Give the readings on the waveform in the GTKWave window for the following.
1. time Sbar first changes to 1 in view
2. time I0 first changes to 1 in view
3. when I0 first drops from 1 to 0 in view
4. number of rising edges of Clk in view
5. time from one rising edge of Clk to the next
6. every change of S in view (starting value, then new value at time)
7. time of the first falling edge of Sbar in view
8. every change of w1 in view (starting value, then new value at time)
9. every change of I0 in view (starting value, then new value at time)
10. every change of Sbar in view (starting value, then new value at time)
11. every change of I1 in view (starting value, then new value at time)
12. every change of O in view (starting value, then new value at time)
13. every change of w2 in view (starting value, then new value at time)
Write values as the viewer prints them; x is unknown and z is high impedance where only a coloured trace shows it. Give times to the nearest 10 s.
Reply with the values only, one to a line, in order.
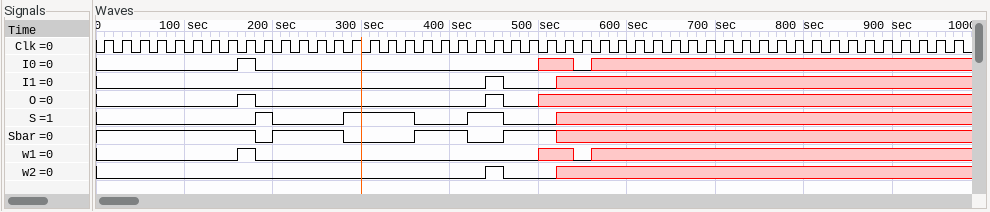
200 s
160 s
180 s
49
20 s
0, 1 at 180 s, 0 at 200 s, 1 at 280 s, 0 at 360 s, 1 at 420 s, 0 at 460 s, x at 520 s
180 s
0, 1 at 160 s, 0 at 180 s, x at 500 s, 0 at 540 s, x at 560 s
0, 1 at 160 s, 0 at 180 s, x at 500 s, 0 at 540 s, x at 560 s
1, 0 at 180 s, 1 at 200 s, 0 at 280 s, 1 at 360 s, 0 at 420 s, 1 at 460 s, x at 520 s
0, 1 at 440 s, 0 at 460 s, x at 520 s
0, 1 at 160 s, 0 at 180 s, 1 at 440 s, 0 at 460 s, x at 500 s
0, 1 at 440 s, 0 at 460 s, x at 520 s
